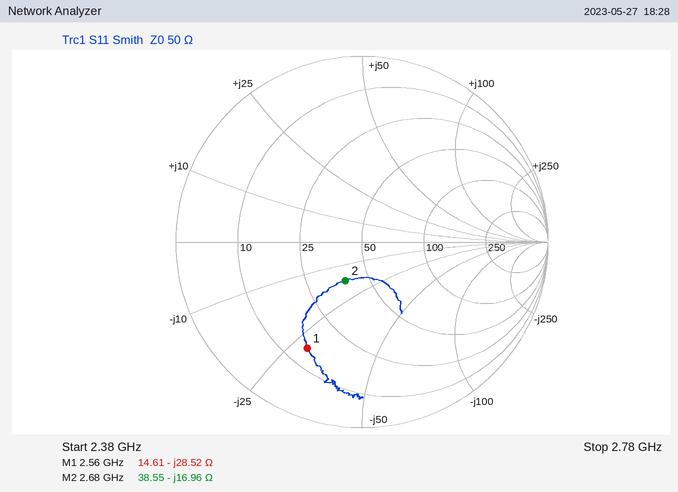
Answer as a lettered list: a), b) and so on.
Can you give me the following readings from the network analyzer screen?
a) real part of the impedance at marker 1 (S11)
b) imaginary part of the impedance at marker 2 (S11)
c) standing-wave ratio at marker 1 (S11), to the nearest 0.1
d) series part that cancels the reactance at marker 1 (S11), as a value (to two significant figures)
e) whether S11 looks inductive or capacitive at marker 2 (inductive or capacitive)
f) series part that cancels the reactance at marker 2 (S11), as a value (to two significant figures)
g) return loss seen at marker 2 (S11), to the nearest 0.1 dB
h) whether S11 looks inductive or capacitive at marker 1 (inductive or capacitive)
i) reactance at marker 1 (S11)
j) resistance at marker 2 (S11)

a) 14.61 Ω
b) -16.96 Ω
c) 4.6
d) 1.8 nH
e) capacitive
f) 1.0 nH
g) 12.9 dB
h) capacitive
i) -28.52 Ω
j) 38.55 Ω
